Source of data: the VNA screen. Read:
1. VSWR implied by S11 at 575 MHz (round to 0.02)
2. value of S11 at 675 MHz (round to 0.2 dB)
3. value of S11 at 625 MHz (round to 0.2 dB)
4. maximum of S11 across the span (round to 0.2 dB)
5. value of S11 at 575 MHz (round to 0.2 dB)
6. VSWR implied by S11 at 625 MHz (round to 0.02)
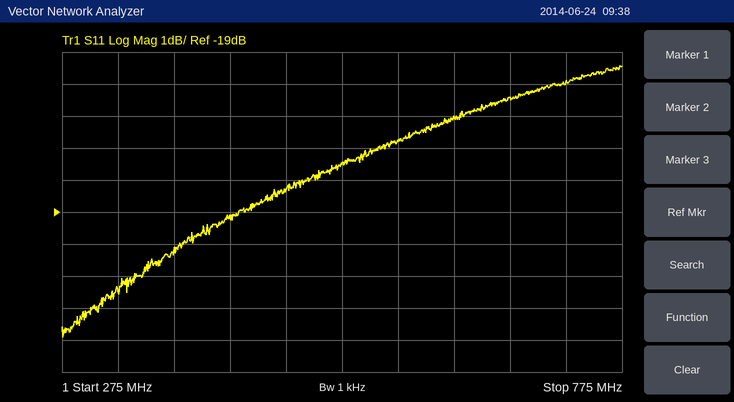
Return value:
1.34
-15.4 dB
-16.0 dB
-14.4 dB
-16.8 dB
1.38
